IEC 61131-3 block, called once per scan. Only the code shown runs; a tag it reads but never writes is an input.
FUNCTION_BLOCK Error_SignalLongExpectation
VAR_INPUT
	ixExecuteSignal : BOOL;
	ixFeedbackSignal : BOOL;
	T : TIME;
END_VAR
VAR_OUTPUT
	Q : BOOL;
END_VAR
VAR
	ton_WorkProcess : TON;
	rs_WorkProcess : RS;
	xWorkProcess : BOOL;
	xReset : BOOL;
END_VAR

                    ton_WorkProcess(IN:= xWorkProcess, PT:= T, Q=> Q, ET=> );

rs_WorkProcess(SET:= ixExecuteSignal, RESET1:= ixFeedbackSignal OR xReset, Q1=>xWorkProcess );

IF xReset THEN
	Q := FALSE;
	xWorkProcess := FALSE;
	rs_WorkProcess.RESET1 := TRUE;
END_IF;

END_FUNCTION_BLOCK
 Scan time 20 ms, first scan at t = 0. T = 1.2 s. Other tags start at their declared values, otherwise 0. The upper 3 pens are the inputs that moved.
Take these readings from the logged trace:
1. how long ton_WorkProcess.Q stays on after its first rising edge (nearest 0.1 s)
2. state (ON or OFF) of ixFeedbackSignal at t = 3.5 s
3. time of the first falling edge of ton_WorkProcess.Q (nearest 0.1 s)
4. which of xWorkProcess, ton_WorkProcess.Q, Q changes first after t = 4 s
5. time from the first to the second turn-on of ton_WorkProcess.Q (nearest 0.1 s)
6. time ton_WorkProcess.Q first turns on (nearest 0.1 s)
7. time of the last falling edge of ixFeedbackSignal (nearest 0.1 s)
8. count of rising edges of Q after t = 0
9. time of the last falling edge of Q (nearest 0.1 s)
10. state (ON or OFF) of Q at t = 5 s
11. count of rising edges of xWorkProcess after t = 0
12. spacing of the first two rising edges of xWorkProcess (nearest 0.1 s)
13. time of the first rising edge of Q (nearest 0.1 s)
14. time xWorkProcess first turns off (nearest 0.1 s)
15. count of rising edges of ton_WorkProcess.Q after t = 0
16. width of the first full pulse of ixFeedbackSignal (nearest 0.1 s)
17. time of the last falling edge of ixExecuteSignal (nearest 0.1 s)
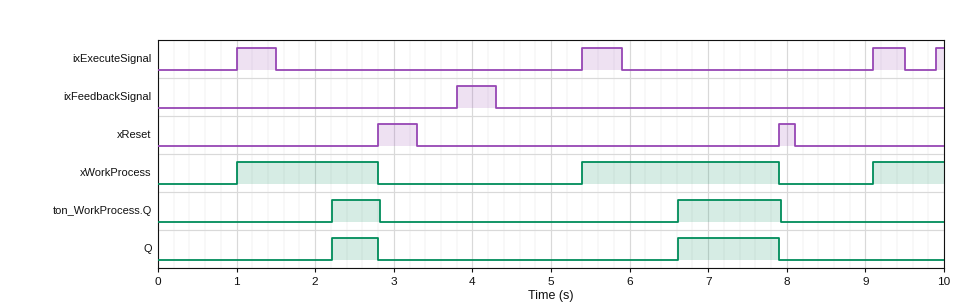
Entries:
0.6 s
OFF
2.8 s
xWorkProcess
4.4 s
2.2 s
4.3 s
2
7.9 s
OFF
3
4.4 s
2.2 s
2.8 s
2
0.5 s
9.5 s
